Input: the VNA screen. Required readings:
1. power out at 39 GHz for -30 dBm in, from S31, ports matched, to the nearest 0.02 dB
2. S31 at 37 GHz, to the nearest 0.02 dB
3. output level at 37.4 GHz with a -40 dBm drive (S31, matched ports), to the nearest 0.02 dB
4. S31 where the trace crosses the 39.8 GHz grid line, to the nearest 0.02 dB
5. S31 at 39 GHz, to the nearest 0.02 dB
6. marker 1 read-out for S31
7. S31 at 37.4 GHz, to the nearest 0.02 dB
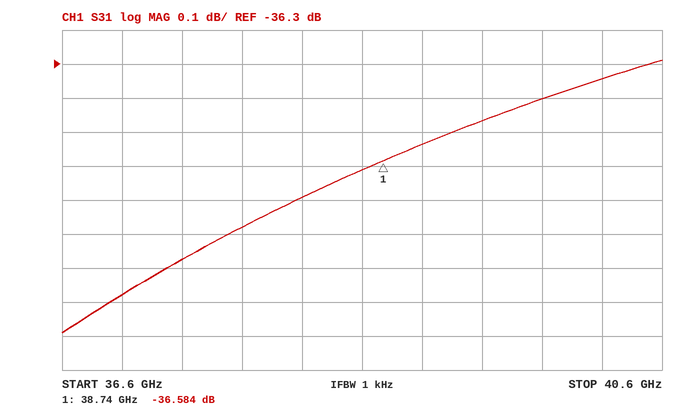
-66.54 dBm
-36.98 dB
-76.88 dBm
-36.40 dB
-36.54 dB
-36.584 dB
-36.88 dB
